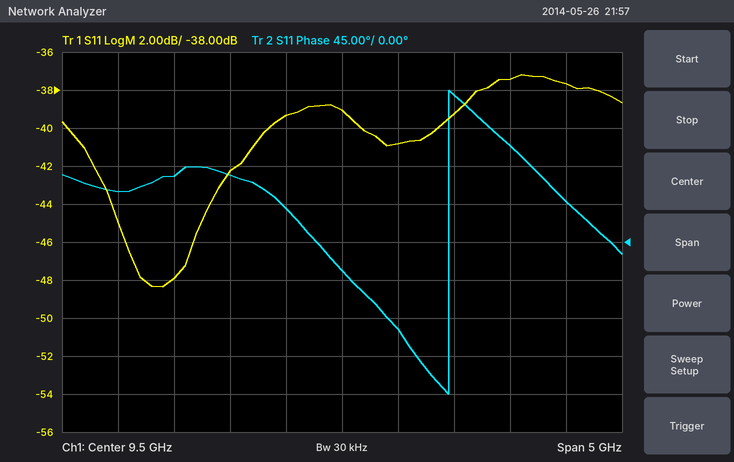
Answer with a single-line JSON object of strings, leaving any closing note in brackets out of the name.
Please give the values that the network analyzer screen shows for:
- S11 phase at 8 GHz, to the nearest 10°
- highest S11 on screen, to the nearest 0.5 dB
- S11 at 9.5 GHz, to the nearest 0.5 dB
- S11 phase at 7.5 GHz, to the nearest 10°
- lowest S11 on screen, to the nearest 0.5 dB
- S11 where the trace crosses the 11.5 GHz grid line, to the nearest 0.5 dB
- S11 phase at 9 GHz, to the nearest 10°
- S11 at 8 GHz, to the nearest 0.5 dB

{"S11 phase at 8 GHz, to the nearest 10°": "80°", "highest S11 on screen, to the nearest 0.5 dB": "-37.0 dB", "S11 at 9.5 GHz, to the nearest 0.5 dB": "-39.0 dB", "S11 phase at 7.5 GHz, to the nearest 10°": "60°", "lowest S11 on screen, to the nearest 0.5 dB": "-48.5 dB", "S11 where the trace crosses the 11.5 GHz grid line, to the nearest 0.5 dB": "-37.5 dB", "S11 phase at 9 GHz, to the nearest 10°": "40°", "S11 at 8 GHz, to the nearest 0.5 dB": "-48.0 dB"}
